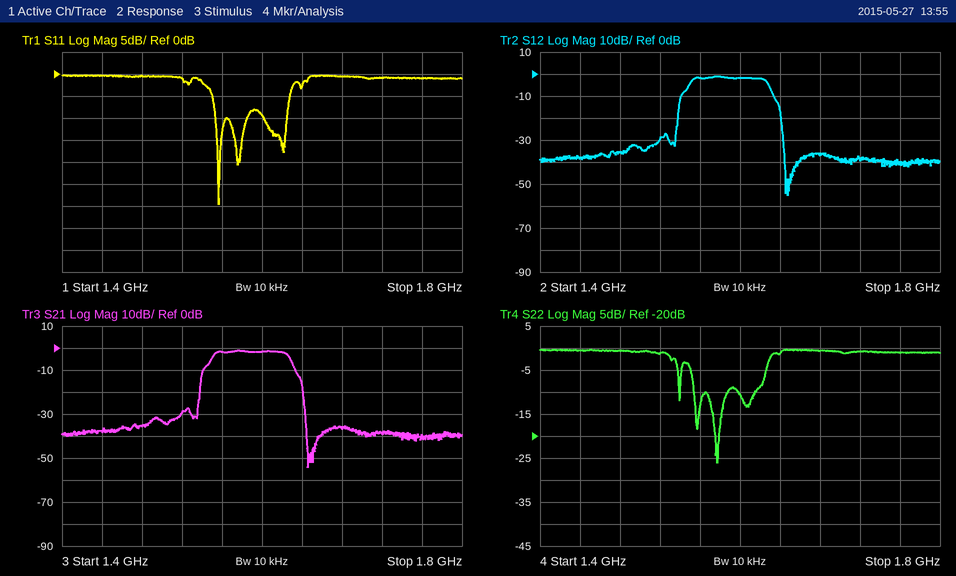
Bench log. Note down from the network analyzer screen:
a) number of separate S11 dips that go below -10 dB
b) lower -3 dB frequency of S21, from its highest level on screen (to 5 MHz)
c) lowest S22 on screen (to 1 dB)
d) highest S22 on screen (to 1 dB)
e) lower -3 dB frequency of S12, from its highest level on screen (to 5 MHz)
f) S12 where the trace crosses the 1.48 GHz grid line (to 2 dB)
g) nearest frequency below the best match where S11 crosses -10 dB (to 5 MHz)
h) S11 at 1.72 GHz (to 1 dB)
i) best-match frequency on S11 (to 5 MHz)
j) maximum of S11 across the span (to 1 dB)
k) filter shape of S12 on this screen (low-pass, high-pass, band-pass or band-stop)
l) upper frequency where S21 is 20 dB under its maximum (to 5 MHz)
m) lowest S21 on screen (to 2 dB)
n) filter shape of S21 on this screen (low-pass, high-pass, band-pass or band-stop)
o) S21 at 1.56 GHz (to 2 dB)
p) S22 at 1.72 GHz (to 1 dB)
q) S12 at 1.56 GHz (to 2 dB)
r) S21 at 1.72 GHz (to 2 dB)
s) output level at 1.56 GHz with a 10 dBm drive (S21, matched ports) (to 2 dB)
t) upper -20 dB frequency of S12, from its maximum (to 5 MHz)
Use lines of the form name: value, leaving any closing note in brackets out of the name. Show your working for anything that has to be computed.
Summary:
number of separate S11 dips that go below -10 dB: 3
lower -3 dB frequency of S21, from its highest level on screen: 1.550 GHz
lowest S22 on screen: -26 dB
highest S22 on screen: 0 dB
lower -3 dB frequency of S12, from its highest level on screen: 1.550 GHz
S12 where the trace crosses the 1.48 GHz grid line: -36 dB
nearest frequency below the best match where S11 crosses -10 dB: 1.555 GHz
S11 at 1.72 GHz: -1 dB
best-match frequency on S11: 1.555 GHz
maximum of S11 across the span: 0 dB
filter shape of S12 on this screen: band-pass
upper frequency where S21 is 20 dB under its maximum: 1.640 GHz
lowest S21 on screen: -54 dB
filter shape of S21 on this screen: band-pass
S21 at 1.56 GHz: -2 dB
S22 at 1.72 GHz: -1 dB
S12 at 1.56 GHz: -2 dB
S21 at 1.72 GHz: -38 dB
output level at 1.56 GHz with a 10 dBm drive (S21, matched ports): 10 dBm + (-2 dB) = 8 dBm
upper -20 dB frequency of S12, from its maximum: 1.640 GHz
